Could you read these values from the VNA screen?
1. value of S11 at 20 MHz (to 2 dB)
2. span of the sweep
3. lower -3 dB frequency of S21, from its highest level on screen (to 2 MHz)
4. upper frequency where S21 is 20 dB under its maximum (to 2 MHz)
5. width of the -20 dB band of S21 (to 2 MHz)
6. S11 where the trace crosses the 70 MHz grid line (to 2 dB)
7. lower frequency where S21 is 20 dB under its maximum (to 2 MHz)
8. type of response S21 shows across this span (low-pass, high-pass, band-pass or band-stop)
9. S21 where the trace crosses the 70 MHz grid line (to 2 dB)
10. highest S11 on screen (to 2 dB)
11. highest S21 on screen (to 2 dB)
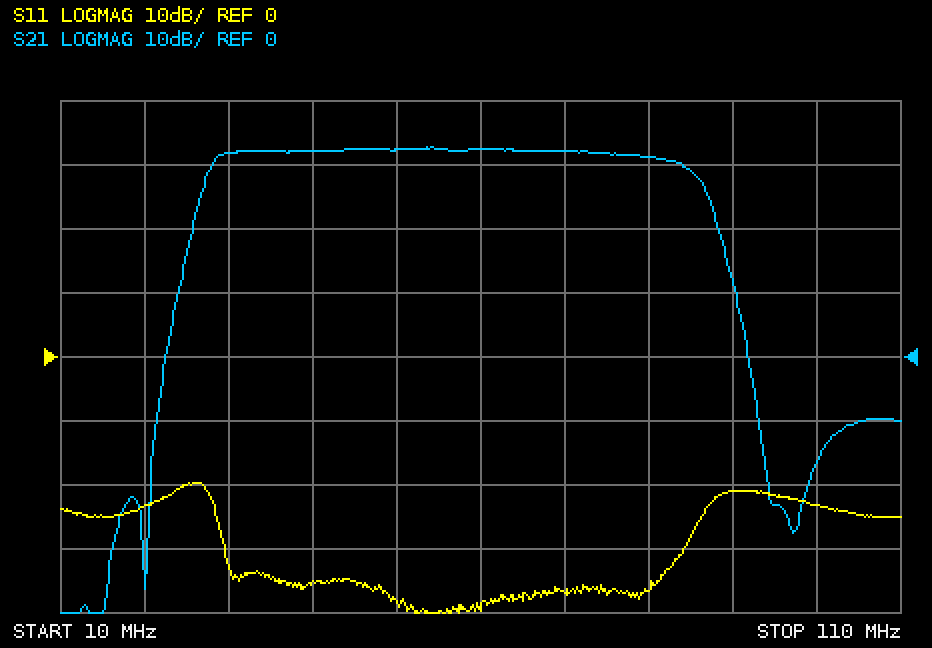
-24 dB
100 MHz
28 MHz
90 MHz
66 MHz
-36 dB
24 MHz
band-pass
32 dB
-20 dB
32 dB
